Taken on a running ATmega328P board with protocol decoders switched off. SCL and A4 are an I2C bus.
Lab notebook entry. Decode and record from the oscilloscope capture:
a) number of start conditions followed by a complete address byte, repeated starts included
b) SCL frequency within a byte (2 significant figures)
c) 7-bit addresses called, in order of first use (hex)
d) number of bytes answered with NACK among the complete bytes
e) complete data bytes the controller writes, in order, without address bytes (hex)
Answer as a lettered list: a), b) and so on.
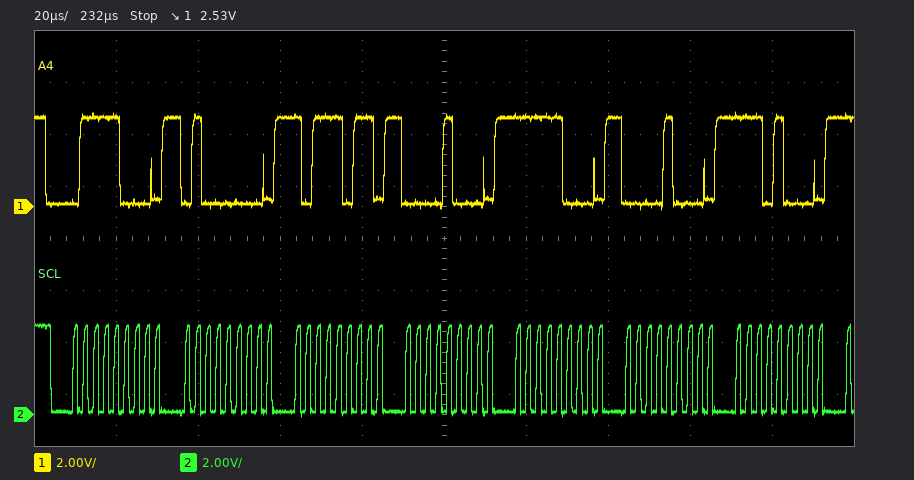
a) 1
b) 400 kHz
c) 0x3C
d) 0
e) 40 BB 08 F8 08 E8
